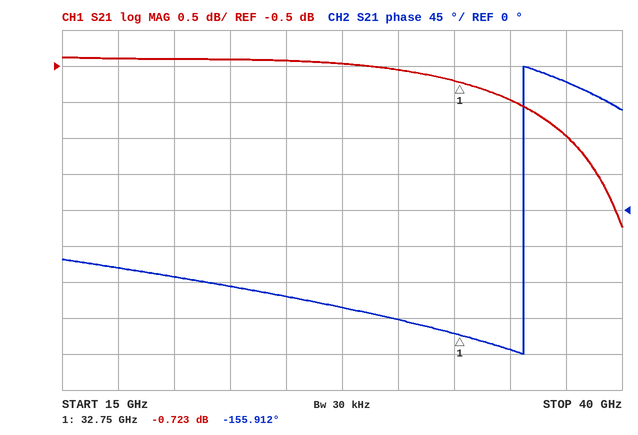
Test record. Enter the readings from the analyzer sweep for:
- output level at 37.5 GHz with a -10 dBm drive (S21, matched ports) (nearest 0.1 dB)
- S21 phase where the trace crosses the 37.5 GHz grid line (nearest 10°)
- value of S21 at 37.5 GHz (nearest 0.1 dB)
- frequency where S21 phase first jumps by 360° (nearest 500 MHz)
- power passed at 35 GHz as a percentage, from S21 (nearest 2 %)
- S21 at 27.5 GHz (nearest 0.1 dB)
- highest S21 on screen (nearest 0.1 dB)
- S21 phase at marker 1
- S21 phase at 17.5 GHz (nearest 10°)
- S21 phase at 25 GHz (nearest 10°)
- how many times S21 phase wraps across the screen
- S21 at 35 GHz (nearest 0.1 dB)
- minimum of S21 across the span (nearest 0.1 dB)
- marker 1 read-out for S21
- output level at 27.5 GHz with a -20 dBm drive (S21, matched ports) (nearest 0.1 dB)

-11.5 dBm
160°
-1.5 dB
35.5 GHz
80 %
-0.5 dB
-0.4 dB
-155.912°
-70°
-110°
1
-1.0 dB
-2.7 dB
-0.723 dB
-20.5 dBm
